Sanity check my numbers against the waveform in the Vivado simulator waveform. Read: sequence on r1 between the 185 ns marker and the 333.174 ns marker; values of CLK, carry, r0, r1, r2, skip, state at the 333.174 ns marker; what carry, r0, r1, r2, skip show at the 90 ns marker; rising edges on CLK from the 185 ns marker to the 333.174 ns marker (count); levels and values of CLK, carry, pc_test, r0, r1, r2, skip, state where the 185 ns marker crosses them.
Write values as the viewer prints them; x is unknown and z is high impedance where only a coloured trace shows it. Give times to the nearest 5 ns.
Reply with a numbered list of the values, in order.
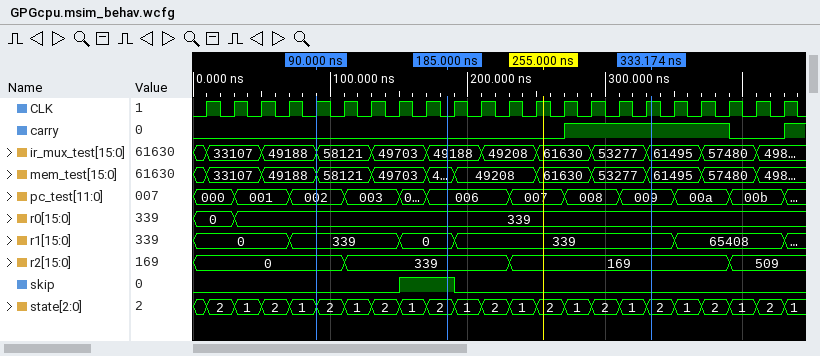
1. 0, 339
2. CLK=1, carry=1, r0=339, r1=339, r2=169, skip=0, state=2
3. carry=0, r0=339, r1=339, r2=0, skip=0
4. 8
5. CLK=0, carry=0, pc_test=006, r0=339, r1=0, r2=339, skip=1, state=2
